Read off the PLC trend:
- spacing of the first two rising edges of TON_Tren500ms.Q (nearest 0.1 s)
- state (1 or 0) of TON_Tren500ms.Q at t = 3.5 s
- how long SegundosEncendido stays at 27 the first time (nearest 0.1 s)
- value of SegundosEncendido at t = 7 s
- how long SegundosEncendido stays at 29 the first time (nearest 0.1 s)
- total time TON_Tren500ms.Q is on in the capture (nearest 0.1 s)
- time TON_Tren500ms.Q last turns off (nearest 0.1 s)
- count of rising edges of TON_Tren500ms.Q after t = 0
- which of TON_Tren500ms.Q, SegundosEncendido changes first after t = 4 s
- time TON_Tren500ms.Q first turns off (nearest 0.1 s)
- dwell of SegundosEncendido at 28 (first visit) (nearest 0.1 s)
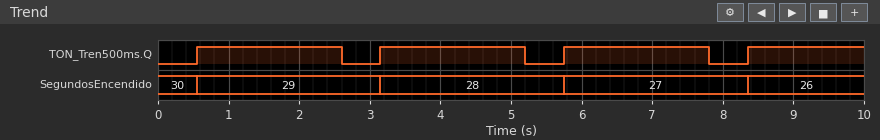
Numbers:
2.6 s
1
2.6 s
27
2.6 s
7.8 s
7.8 s
4
TON_Tren500ms.Q
2.6 s
2.6 s
